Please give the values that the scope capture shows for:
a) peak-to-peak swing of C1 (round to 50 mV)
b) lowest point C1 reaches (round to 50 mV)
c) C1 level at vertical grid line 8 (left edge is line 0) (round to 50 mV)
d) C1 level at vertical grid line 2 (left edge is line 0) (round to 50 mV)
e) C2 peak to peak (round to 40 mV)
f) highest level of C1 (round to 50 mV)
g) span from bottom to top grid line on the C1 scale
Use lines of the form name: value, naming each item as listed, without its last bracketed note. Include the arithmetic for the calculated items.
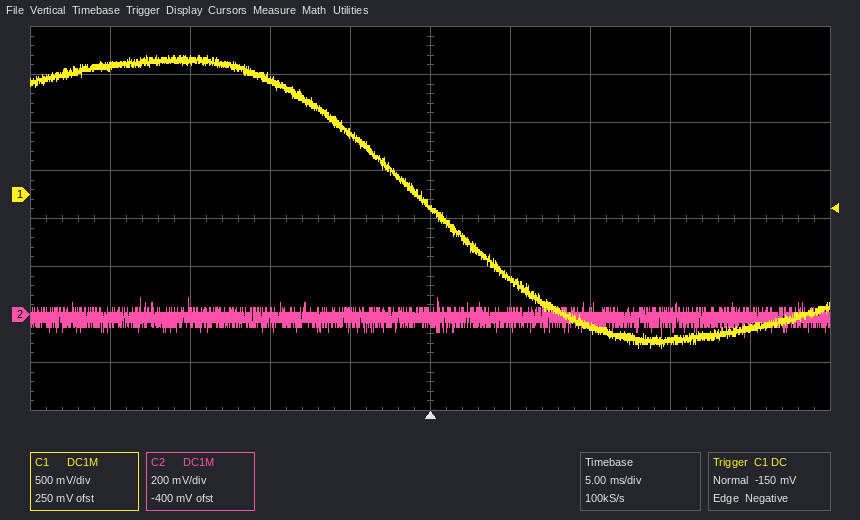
peak-to-peak swing of C1: 1.45 V − (-1.60 V) = 3.05 V
lowest point C1 reaches: -1.60 V
C1 level at vertical grid line 8 (left edge is line 0): -1.50 V
C1 level at vertical grid line 2 (left edge is line 0): 1.40 V
C2 peak to peak: 160 mV
highest level of C1: 1.45 V
span from bottom to top grid line on the C1 scale: 4 V
